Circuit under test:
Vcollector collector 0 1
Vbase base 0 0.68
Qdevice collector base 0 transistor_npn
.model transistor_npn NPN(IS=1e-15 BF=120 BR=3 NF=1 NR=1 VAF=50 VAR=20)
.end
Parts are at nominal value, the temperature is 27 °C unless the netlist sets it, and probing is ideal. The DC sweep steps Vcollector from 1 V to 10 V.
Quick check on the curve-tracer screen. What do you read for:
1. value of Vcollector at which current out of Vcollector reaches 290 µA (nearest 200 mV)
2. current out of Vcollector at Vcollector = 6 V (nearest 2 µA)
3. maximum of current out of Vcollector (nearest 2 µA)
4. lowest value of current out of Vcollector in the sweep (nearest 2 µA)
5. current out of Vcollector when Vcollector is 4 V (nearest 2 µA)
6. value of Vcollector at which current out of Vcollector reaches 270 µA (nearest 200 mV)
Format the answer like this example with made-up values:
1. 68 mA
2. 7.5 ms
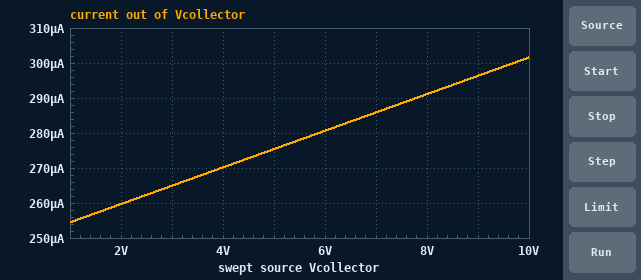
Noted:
1. 7.8 V
2. 280 µA
3. 302 µA
4. 254 µA
5. 270 µA
6. 4.0 V
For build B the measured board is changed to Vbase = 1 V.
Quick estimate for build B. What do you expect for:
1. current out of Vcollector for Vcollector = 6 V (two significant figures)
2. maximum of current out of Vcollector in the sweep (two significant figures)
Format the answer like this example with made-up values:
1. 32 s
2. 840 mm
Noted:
1. 65 A
2. 70 A
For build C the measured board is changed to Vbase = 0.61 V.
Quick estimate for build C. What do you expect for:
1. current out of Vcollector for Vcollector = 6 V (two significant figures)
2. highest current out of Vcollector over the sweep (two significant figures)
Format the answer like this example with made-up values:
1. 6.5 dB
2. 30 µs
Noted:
1. 19 µA
2. 20 µA
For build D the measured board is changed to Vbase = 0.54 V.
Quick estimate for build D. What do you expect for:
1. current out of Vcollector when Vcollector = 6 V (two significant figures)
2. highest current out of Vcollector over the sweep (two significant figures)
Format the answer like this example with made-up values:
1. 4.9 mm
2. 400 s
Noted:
1. 1.3 µA
2. 1.4 µA
